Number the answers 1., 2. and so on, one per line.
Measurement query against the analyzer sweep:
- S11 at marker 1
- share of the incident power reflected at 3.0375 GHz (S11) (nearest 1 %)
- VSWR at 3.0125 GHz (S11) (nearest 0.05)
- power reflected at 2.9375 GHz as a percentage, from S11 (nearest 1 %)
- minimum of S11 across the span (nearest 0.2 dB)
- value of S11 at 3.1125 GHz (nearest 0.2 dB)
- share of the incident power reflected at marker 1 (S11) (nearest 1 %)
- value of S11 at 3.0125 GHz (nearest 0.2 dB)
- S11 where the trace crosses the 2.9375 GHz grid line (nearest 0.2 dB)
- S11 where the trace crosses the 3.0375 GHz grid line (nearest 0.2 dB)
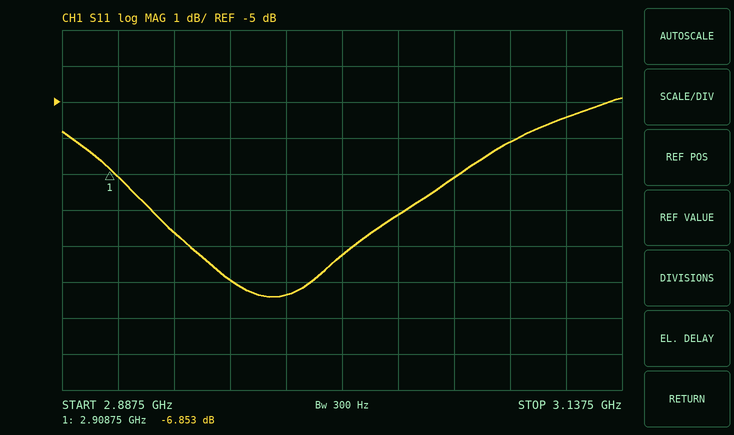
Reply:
1. -6.853 dB
2. 15 %
3. 2.05
4. 14 %
5. -10.4 dB
6. -5.4 dB
7. 21 %
8. -9.2 dB
9. -8.6 dB
10. -8.2 dB
